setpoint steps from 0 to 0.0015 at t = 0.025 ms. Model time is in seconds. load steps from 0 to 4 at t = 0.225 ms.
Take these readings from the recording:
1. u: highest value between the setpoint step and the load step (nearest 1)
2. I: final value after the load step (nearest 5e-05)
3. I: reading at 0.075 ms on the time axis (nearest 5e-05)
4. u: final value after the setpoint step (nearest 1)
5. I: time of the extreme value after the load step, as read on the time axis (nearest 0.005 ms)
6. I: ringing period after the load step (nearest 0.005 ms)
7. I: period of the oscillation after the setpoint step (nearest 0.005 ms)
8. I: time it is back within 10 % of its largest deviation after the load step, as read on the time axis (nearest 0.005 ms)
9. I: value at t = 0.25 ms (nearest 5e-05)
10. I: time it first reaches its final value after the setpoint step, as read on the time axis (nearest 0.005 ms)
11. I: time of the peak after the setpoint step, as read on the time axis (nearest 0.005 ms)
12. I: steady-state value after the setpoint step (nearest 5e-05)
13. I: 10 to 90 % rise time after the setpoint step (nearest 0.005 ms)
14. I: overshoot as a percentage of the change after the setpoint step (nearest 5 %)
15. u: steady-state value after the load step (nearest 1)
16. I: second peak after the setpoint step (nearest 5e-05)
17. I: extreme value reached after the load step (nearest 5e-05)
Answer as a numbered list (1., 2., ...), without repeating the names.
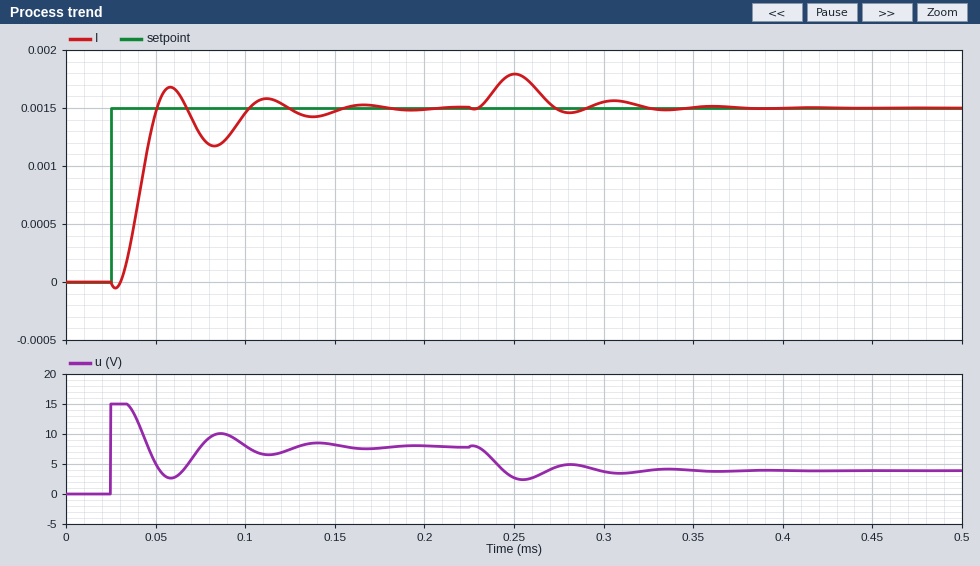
1. 15
2. 0.00150
3. 0.00125
4. 8
5. 0.250 ms
6. 0.055 ms
7. 0.055 ms
8. 0.320 ms
9. 0.00180
10. 0.050 ms
11. 0.060 ms
12. 0.00150
13. 0.015 ms
14. 10 %
15. 4
16. 0.00160
17. 0.00180
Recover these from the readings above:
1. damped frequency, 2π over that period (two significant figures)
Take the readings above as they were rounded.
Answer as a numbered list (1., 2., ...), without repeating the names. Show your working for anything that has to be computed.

1. 2π / 0.055 = 110 rad/ms
